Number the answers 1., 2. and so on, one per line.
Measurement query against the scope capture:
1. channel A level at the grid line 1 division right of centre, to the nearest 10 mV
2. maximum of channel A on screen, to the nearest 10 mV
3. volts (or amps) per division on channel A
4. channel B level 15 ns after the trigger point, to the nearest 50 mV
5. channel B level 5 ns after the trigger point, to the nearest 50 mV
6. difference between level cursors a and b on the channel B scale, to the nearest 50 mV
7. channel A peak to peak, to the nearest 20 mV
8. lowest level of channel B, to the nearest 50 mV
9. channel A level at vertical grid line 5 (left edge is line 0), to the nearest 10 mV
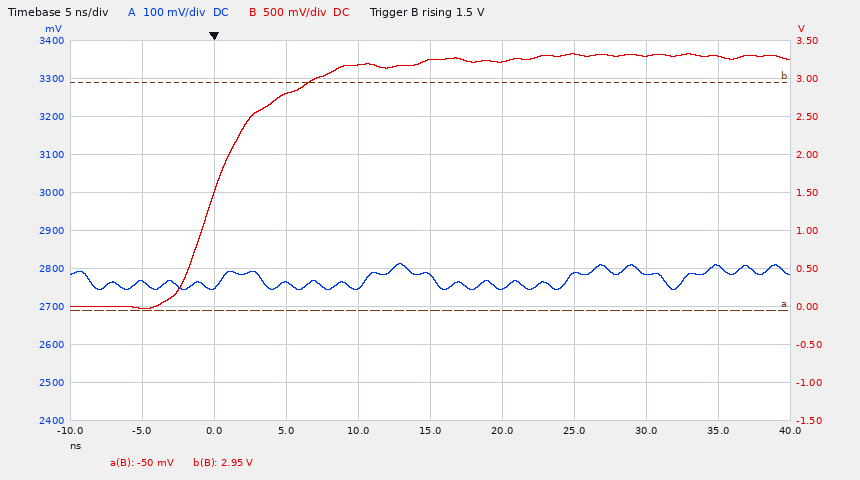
1. 2.75 V
2. 2.81 V
3. 100 mV
4. 3.25 V
5. 2.80 V
6. 3.00 V
7. 60 mV
8. -50 mV
9. 2.78 V
